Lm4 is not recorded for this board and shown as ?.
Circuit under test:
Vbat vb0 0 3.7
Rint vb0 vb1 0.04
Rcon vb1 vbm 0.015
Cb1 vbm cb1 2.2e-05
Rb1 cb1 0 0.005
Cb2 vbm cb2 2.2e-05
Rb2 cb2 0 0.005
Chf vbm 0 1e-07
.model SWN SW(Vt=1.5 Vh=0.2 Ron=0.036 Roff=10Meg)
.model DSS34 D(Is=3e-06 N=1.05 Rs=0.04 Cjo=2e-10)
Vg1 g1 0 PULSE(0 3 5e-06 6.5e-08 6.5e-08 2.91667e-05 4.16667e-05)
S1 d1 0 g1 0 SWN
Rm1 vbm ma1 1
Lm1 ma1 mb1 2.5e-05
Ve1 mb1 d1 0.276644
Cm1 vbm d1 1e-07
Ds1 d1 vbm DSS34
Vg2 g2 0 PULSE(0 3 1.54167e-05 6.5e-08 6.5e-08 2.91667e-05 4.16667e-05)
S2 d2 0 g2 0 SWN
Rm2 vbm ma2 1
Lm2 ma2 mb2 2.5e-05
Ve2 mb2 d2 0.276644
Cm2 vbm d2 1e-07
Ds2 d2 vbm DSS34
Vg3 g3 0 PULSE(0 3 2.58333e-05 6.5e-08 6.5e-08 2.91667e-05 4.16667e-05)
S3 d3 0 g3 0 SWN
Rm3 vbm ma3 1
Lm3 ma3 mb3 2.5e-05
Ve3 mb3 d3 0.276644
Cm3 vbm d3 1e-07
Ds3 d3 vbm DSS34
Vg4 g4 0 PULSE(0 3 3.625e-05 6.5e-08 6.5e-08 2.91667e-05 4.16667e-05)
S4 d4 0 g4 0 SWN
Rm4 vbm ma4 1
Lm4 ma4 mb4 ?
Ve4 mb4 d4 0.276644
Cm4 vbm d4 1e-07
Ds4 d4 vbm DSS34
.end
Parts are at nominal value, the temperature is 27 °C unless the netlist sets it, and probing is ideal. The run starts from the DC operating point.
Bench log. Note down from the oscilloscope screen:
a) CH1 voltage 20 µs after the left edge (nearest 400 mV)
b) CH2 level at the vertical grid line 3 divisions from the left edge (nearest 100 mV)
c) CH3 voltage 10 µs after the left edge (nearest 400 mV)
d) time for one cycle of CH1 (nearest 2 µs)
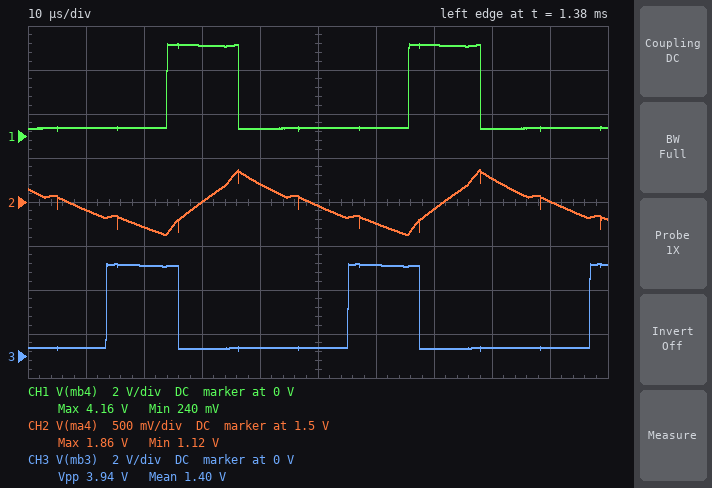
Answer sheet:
400 mV
1.5 V
400 mV
42 µs
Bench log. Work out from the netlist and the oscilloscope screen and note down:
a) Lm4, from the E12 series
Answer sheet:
47 µH
